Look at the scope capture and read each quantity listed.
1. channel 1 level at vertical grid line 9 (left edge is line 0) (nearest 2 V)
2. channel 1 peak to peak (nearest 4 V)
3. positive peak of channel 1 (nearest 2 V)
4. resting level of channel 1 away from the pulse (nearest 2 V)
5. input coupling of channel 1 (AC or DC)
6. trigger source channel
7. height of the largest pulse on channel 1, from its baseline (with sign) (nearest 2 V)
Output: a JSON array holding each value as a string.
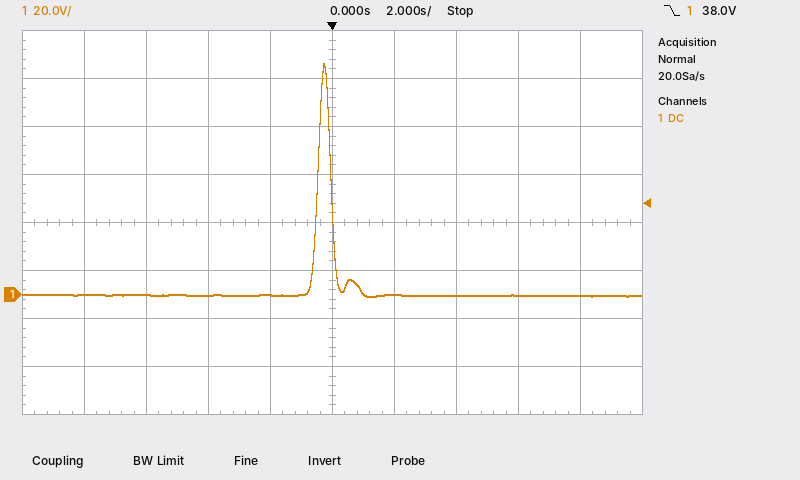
["0 V", "96 V", "96 V", "0 V", "DC", "channel 1", "+96 V"]
